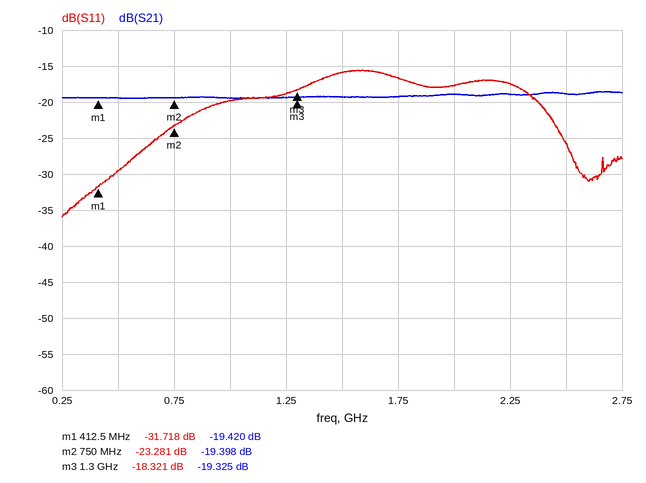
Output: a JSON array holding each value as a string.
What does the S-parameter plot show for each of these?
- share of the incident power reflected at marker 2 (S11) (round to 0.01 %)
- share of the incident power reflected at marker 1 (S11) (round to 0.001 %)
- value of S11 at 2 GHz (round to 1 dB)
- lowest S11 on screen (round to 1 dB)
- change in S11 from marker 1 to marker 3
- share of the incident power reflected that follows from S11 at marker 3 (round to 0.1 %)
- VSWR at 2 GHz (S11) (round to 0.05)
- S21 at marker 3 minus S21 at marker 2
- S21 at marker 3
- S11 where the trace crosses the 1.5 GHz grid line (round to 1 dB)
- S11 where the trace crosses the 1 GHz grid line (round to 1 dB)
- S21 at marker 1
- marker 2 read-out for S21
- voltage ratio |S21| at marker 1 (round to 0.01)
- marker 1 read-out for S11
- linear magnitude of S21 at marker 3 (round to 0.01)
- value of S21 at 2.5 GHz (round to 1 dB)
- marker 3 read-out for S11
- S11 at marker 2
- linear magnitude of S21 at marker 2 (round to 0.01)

["0.47 %", "0.067 %", "-18 dB", "-36 dB", "13.397 dB", "1.5 %", "1.30", "0.073 dB", "-19.325 dB", "-16 dB", "-20 dB", "-19.420 dB", "-19.398 dB", "0.11", "-31.718 dB", "0.11", "-19 dB", "-18.321 dB", "-23.281 dB", "0.11"]
